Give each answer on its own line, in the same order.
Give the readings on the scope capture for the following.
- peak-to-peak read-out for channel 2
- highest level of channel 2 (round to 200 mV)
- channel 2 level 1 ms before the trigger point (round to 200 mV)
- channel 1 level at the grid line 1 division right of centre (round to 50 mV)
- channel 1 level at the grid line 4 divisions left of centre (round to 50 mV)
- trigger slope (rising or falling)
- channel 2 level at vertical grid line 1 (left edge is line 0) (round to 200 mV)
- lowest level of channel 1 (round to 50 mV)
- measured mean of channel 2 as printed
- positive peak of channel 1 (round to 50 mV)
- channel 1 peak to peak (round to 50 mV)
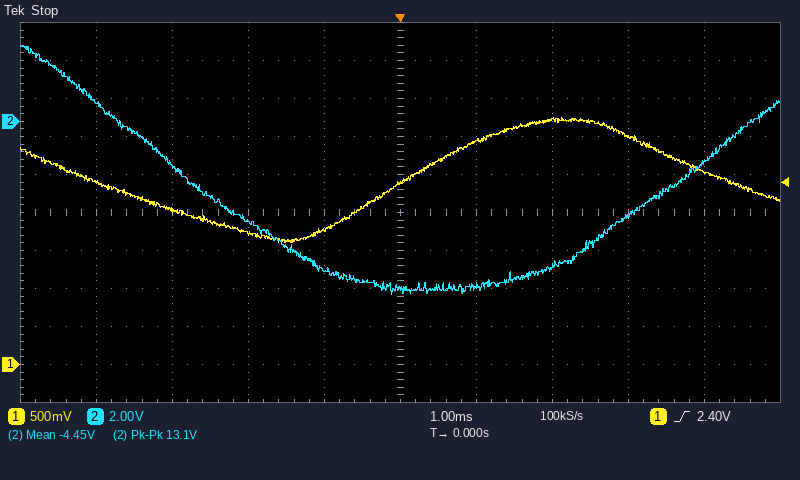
13.1 V
4.0 V
-7.8 V
2.95 V
2.40 V
rising
1.0 V
1.60 V
-4.45 V
3.25 V
1.65 V
